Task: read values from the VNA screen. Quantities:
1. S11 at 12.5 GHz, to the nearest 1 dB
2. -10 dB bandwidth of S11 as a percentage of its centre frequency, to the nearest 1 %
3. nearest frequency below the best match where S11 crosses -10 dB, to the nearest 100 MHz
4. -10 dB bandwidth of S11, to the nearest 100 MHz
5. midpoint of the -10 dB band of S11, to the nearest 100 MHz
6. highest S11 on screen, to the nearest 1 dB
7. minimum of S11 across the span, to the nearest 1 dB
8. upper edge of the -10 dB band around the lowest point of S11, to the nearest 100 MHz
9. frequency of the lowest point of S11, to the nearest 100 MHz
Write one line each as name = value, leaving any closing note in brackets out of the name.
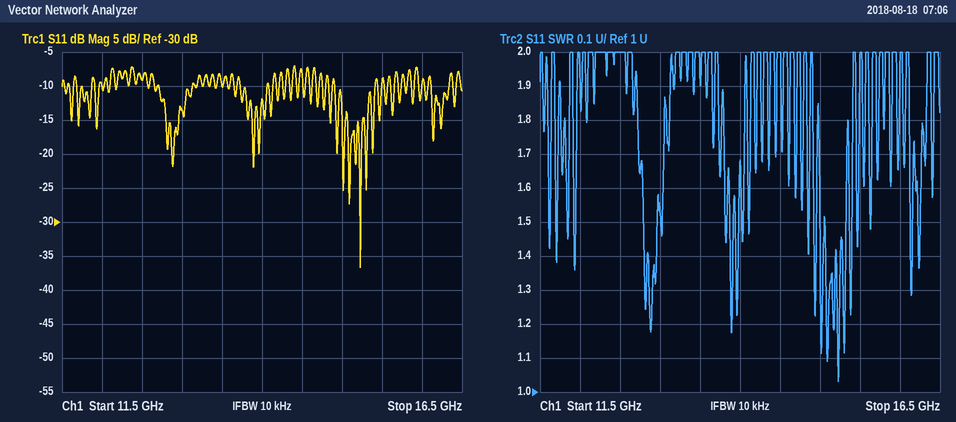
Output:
S11 at 12.5 GHz, to the nearest 1 dB = -9 dB
-10 dB bandwidth of S11 as a percentage of its centre frequency, to the nearest 1 % = 3 %
nearest frequency below the best match where S11 crosses -10 dB, to the nearest 100 MHz = 14.9 GHz
-10 dB bandwidth of S11, to the nearest 100 MHz = 500 MHz
midpoint of the -10 dB band of S11, to the nearest 100 MHz = 15.2 GHz
highest S11 on screen, to the nearest 1 dB = -7 dB
minimum of S11 across the span, to the nearest 1 dB = -37 dB
upper edge of the -10 dB band around the lowest point of S11, to the nearest 100 MHz = 15.4 GHz
frequency of the lowest point of S11, to the nearest 100 MHz = 15.2 GHz
